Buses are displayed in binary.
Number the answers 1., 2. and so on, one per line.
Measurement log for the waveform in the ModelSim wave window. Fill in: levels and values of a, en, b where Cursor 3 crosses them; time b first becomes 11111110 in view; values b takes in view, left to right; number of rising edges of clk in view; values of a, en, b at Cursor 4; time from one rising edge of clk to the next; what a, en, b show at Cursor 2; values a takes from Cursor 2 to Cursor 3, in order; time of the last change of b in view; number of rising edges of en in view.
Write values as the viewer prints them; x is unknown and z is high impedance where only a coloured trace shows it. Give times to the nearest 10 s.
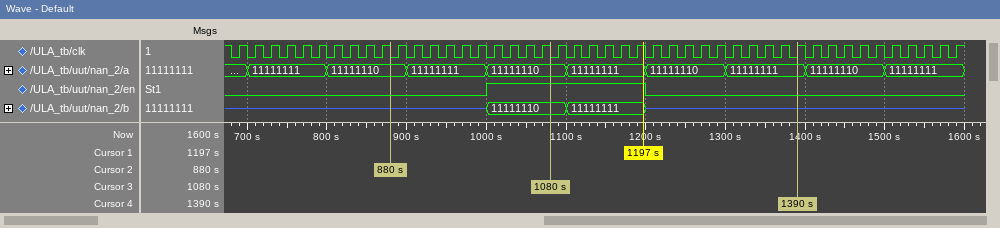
1. a=11111110, en=1, b=11111110
2. 1000 s
3. z, 11111110, 11111111, z
4. 46
5. a=11111111, en=0, b=z
6. 20 s
7. a=11111110, en=0, b=z
8. 11111110, 11111111, 11111110
9. 1200 s
10. 1
